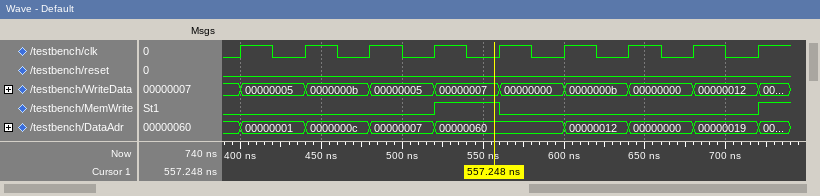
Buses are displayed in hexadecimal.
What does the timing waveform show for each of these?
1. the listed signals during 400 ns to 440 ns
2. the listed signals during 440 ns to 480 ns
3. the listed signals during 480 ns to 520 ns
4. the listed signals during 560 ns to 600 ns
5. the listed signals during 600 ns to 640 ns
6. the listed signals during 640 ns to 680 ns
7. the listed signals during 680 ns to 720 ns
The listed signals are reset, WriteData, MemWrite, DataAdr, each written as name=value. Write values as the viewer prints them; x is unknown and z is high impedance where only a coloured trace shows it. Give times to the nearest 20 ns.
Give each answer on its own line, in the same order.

reset=0, WriteData=00000005, MemWrite=0, DataAdr=00000001
reset=0, WriteData=0000000b, MemWrite=0, DataAdr=0000000c
reset=0, WriteData=00000005, MemWrite=0, DataAdr=00000007
reset=0, WriteData=00000000, MemWrite=0, DataAdr=00000060
reset=0, WriteData=0000000b, MemWrite=0, DataAdr=00000012
reset=0, WriteData=00000000, MemWrite=0, DataAdr=00000000
reset=0, WriteData=00000012, MemWrite=0, DataAdr=00000019
